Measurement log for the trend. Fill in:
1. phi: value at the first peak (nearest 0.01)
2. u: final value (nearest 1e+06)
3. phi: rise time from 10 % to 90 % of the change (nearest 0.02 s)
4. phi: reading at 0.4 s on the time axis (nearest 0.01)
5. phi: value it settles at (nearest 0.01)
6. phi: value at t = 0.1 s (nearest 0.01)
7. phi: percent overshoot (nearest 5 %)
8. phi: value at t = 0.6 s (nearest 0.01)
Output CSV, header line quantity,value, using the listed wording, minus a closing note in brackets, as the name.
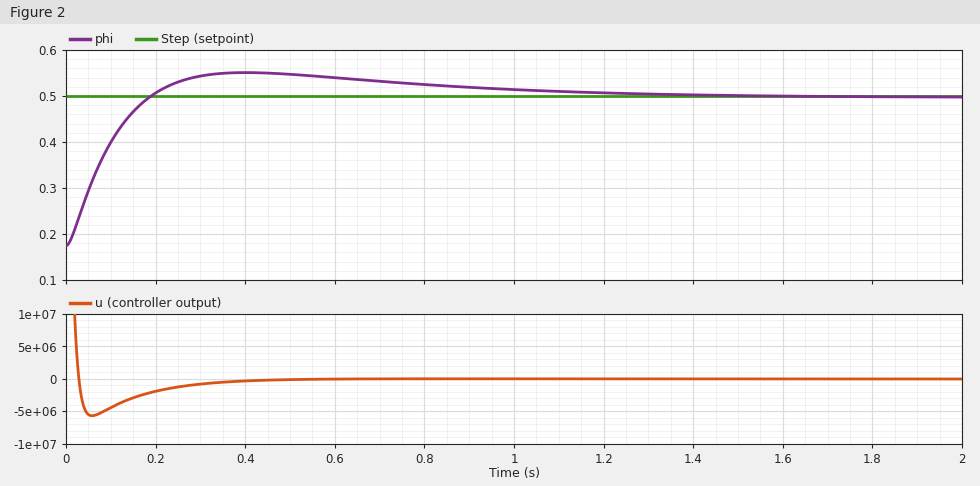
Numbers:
quantity,value
phi: value at the first peak,0.55
u: final value,0
phi: rise time from 10 % to 90 % of the change,0.14 s
phi: reading at 0.4 s on the time axis,0.55
phi: value it settles at,0.50
phi: value at t = 0.1 s,0.40
phi: percent overshoot,15 %
phi: value at t = 0.6 s,0.54
